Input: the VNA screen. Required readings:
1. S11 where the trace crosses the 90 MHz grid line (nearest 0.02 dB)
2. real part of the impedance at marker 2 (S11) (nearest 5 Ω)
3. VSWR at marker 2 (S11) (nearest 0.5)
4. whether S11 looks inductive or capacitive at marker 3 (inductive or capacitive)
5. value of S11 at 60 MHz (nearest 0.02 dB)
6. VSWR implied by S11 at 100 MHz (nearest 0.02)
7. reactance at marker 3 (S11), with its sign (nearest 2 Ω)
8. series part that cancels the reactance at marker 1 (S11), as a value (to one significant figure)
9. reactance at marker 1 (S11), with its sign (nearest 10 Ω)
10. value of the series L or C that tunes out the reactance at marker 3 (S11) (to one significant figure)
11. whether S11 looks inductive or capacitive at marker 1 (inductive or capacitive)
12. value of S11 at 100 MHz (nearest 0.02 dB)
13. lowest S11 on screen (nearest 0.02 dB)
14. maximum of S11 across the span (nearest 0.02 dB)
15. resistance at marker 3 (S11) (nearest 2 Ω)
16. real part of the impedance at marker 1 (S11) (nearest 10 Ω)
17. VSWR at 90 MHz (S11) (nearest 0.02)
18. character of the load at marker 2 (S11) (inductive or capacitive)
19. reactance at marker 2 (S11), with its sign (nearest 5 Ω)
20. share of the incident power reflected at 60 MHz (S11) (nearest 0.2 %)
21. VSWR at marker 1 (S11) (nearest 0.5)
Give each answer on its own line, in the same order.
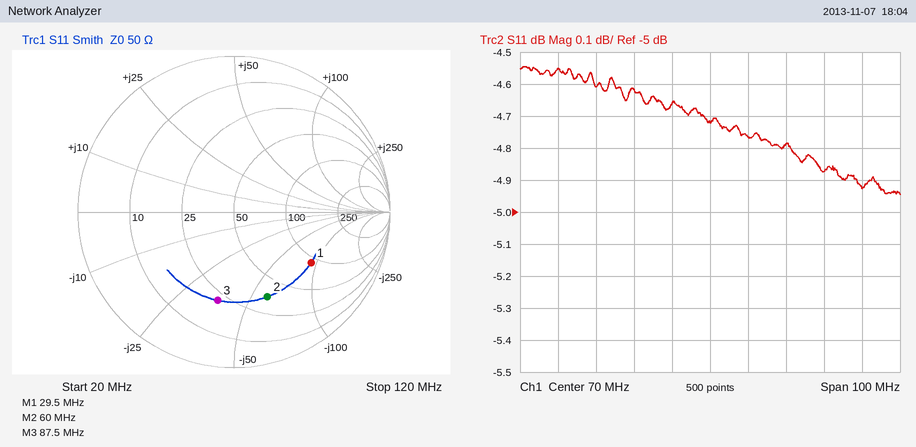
-4.78 dB
35 Ω
4.0
capacitive
-4.66 dB
3.66
-36 Ω
500 nH
-90 Ω
70 nH
capacitive
-4.88 dB
-4.94 dB
-4.54 dB
22 Ω
90 Ω
3.72
capacitive
-60 Ω
34.2 %
4.0
